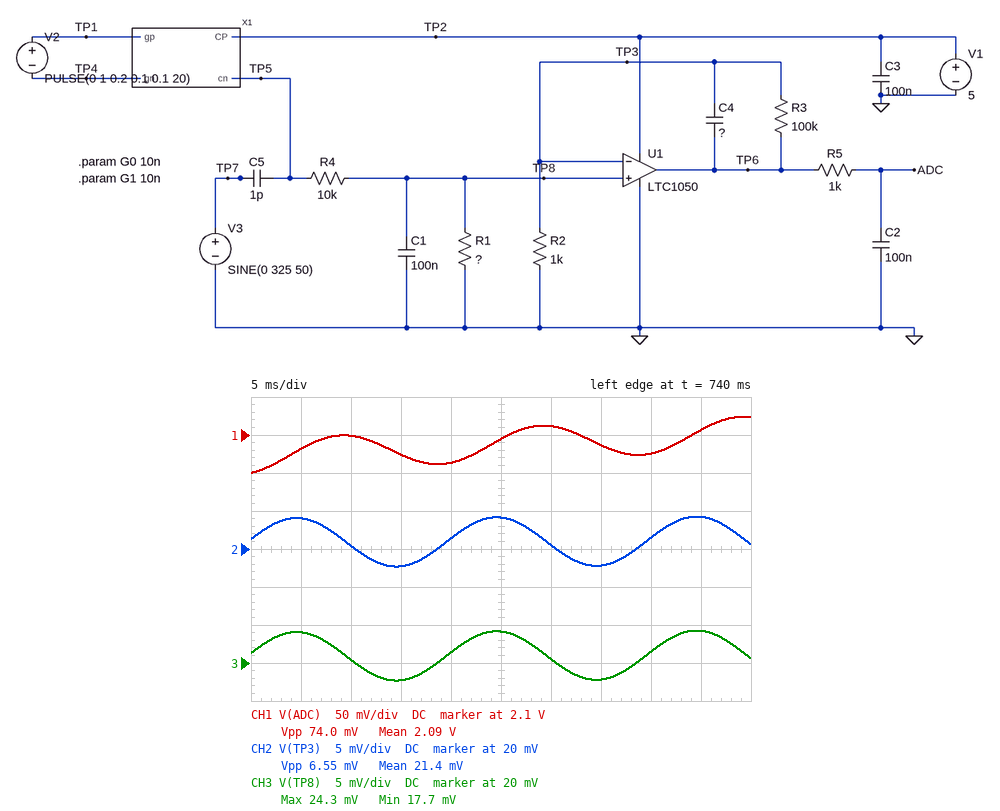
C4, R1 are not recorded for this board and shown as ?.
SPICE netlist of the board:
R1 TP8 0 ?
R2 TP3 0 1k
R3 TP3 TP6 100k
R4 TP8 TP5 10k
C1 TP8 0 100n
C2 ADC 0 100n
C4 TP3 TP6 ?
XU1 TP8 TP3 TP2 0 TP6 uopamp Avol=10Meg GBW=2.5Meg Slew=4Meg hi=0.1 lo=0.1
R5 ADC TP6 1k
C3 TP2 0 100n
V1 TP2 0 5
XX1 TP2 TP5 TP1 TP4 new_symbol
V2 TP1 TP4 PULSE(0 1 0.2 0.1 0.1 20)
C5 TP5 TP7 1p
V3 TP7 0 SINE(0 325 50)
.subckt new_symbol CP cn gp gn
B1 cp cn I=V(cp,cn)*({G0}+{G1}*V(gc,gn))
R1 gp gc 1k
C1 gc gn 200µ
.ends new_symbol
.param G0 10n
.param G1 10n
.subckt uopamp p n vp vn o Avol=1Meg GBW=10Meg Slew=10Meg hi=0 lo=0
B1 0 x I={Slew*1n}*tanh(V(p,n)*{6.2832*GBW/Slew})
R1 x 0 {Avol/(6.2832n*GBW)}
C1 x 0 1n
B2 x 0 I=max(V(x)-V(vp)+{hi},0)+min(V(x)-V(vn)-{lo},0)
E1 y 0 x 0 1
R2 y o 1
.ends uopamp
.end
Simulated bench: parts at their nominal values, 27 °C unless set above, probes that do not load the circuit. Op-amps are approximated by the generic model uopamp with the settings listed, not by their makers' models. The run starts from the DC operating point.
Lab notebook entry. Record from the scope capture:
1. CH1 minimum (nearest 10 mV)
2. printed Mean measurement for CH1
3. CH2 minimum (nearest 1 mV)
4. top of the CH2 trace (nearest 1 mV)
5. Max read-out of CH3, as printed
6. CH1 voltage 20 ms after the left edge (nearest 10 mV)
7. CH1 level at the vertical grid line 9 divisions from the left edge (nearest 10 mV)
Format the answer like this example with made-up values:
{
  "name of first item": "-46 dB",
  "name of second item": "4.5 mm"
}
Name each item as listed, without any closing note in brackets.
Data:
{
  "CH1 minimum": "2.05 V",
  "printed Mean measurement for CH1": "2.09 V",
  "CH2 minimum": "18 mV",
  "top of the CH2 trace": "24 mV",
  "Max read-out of CH3, as printed": "24.3 mV",
  "CH1 voltage 20 ms after the left edge": "2.06 V",
  "CH1 level at the vertical grid line 9 divisions from the left edge": "2.11 V"
}
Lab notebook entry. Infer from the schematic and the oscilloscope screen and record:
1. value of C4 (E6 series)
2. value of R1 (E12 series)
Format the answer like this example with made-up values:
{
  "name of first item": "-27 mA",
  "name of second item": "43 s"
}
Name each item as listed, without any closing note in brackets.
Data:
{
  "value of C4": "470 nF",
  "value of R1": "220 kΩ"
}
